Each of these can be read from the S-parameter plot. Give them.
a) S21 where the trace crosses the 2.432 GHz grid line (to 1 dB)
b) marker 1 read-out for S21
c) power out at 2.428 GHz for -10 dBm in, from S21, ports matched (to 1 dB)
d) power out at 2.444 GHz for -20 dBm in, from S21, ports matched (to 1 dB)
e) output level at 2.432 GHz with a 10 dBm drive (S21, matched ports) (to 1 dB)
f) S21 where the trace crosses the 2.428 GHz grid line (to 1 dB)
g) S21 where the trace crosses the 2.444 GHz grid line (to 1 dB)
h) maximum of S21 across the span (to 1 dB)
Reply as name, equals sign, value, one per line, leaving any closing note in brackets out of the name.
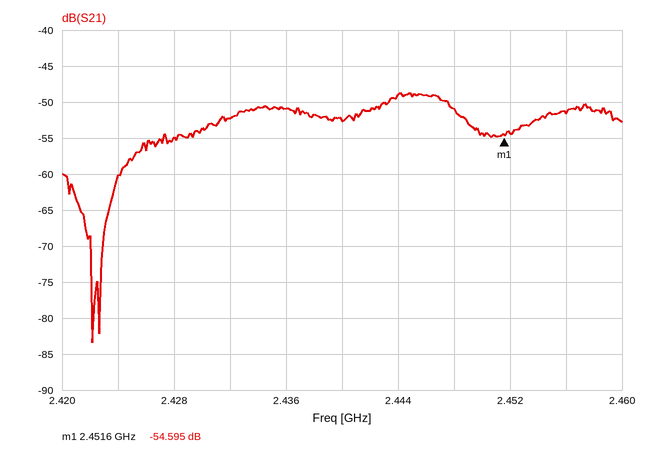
S21 where the trace crosses the 2.432 GHz grid line = -52 dB
marker 1 read-out for S21 = -54.595 dB
power out at 2.428 GHz for -10 dBm in, from S21, ports matched = -65 dBm
power out at 2.444 GHz for -20 dBm in, from S21, ports matched = -69 dBm
output level at 2.432 GHz with a 10 dBm drive (S21, matched ports) = -42 dBm
S21 where the trace crosses the 2.428 GHz grid line = -55 dB
S21 where the trace crosses the 2.444 GHz grid line = -49 dB
maximum of S21 across the span = -49 dB
